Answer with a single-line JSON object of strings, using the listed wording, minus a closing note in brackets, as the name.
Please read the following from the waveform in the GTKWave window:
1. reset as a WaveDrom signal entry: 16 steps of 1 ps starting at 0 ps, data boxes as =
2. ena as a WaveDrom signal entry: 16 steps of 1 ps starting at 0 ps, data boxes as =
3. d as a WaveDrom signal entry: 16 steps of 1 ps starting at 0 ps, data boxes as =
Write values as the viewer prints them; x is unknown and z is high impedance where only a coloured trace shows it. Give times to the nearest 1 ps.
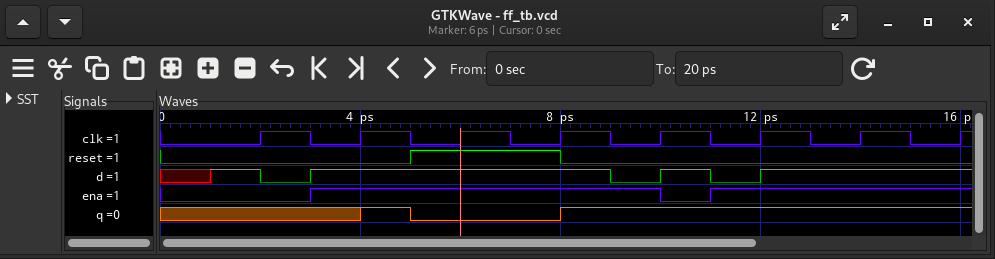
{"reset as a WaveDrom signal entry: 16 steps of 1 ps starting at 0 ps, data boxes as =": "{name: 'reset', wave: '0....1..0.......'}", "ena as a WaveDrom signal entry: 16 steps of 1 ps starting at 0 ps, data boxes as =": "{name: 'ena', wave: '0..1......01....'}", "d as a WaveDrom signal entry: 16 steps of 1 ps starting at 0 ps, data boxes as =": "{name: 'd', wave: 'x101.....0101...'}"}
